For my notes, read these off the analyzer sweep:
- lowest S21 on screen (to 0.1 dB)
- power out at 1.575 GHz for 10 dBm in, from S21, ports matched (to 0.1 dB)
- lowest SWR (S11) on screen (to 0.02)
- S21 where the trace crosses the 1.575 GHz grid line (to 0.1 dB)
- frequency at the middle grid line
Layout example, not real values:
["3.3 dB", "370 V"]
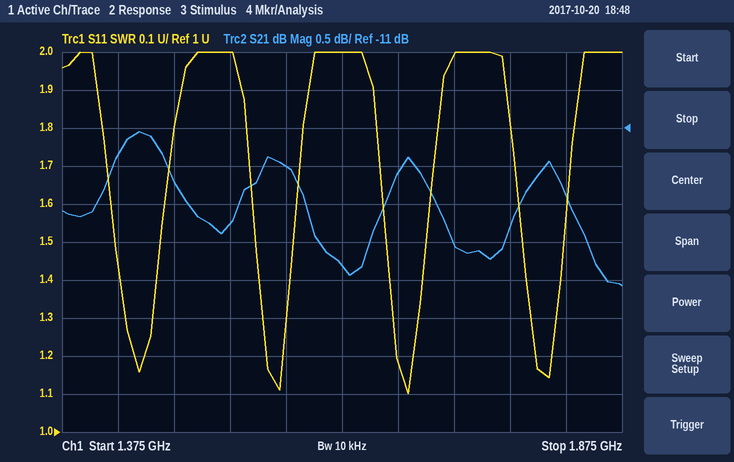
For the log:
["-13.1 dB", "-1.5 dBm", "1.10", "-11.5 dB", "1.625 GHz"]
